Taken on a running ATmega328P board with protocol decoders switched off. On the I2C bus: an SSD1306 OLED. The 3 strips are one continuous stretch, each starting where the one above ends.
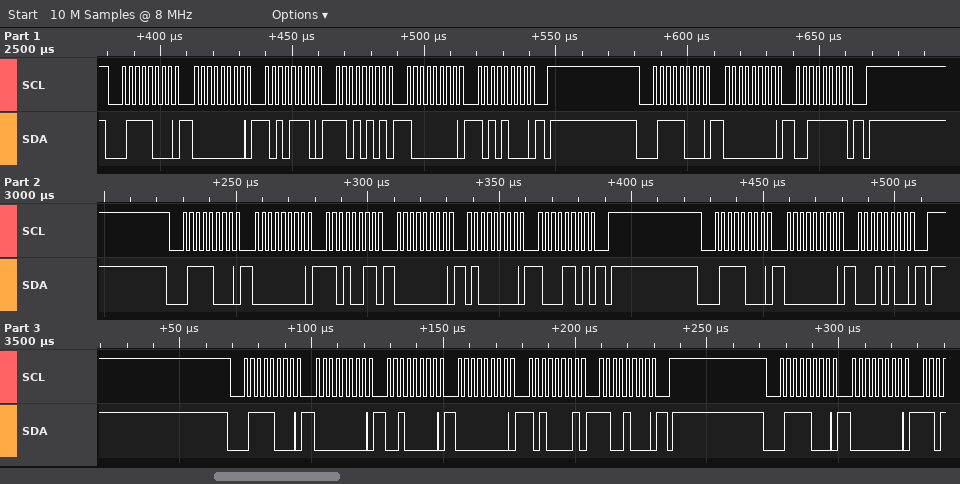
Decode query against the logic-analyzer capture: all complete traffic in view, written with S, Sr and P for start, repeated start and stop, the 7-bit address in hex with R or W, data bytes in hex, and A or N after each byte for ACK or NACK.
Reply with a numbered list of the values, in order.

1. S 3CW A 00 A AE A D5 A 80 A A8 A P S 3CW A 00 A 3F A P S 3CW A 00 A D3 A 00 A 40 A 8D A P S 3CW A 00 A 14 A P S 3CW A 00 A 20 A 00 A A1 A C8 A P S 3CW A 00 A
